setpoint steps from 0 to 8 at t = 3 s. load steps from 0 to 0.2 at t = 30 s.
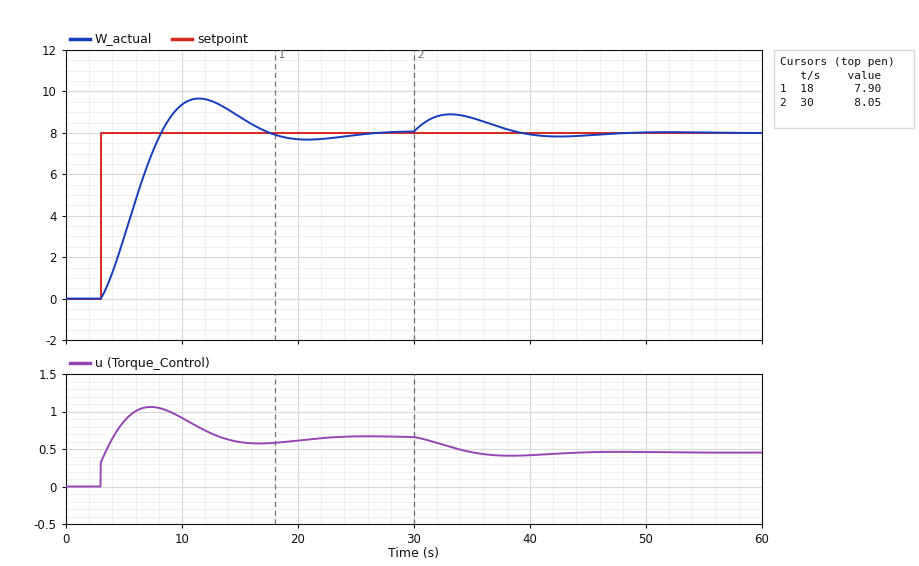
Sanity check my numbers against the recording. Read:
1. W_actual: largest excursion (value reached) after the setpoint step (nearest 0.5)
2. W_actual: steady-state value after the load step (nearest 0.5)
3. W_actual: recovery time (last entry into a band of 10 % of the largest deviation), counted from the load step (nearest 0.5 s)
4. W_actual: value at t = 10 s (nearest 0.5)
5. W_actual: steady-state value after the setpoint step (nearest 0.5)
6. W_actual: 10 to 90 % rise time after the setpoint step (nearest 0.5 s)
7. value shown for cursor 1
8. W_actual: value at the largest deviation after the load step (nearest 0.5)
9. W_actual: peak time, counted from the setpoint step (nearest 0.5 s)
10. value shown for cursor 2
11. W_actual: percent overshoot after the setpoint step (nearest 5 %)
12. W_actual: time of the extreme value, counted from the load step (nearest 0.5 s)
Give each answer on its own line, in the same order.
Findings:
9.5
8.0
16.0 s
9.5
8.0
4.0 s
7.90
9.0
8.5 s
8.05
20 %
3.0 s
